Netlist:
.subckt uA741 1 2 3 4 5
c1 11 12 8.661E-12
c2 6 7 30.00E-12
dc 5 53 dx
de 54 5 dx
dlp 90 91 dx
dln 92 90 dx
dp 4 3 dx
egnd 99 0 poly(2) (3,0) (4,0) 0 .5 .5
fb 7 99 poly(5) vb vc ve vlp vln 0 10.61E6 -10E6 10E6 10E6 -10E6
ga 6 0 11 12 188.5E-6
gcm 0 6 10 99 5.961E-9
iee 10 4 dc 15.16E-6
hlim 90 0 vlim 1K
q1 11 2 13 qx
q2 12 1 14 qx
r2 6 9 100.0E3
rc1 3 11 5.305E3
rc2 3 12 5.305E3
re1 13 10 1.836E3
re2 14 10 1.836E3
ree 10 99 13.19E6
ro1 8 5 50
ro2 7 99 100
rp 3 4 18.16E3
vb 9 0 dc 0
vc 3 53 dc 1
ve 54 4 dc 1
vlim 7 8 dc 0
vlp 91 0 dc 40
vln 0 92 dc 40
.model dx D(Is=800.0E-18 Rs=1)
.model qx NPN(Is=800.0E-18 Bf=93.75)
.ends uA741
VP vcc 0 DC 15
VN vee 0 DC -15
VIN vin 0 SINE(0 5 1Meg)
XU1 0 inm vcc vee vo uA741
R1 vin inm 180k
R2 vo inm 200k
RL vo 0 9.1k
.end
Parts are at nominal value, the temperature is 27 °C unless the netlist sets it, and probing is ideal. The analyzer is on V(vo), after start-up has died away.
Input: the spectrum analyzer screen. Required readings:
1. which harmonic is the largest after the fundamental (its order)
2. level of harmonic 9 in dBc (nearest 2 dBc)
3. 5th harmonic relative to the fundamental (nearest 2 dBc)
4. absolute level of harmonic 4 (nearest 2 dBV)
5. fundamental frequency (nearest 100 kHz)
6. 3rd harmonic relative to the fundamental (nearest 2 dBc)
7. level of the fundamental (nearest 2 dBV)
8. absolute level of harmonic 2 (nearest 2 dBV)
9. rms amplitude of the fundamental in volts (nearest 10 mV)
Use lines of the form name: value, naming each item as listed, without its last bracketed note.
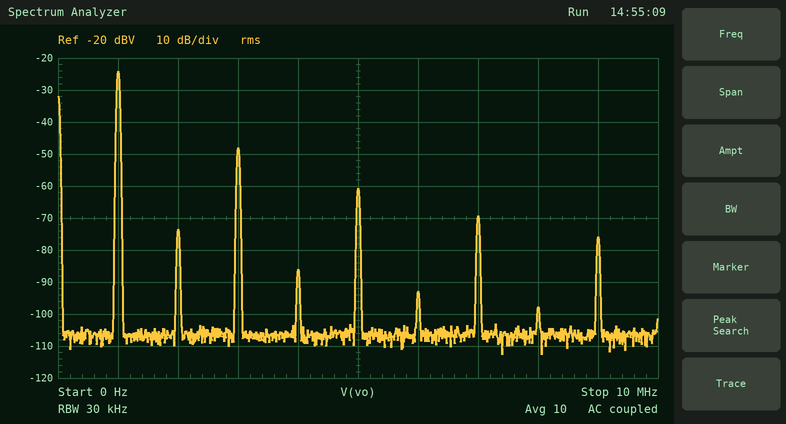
which harmonic is the largest after the fundamental: 3
level of harmonic 9 in dBc: -52 dBc
5th harmonic relative to the fundamental: -36 dBc
absolute level of harmonic 4: -86 dBV
fundamental frequency: 1.0 MHz
3rd harmonic relative to the fundamental: -24 dBc
level of the fundamental: -24 dBV
absolute level of harmonic 2: -74 dBV
rms amplitude of the fundamental in volts: 60 mV
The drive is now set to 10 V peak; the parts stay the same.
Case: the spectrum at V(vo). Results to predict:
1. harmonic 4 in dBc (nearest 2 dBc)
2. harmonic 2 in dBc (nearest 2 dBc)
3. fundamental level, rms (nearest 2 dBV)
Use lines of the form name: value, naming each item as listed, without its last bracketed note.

harmonic 4 in dBc: -56 dBc
harmonic 2 in dBc: -44 dBc
fundamental level, rms: -24 dBV
